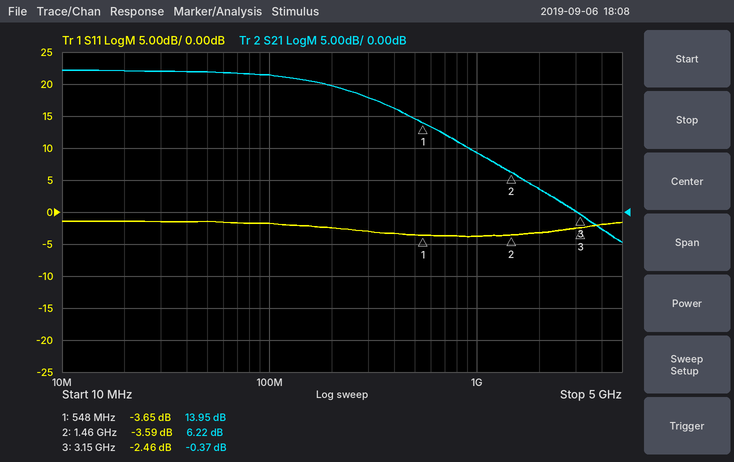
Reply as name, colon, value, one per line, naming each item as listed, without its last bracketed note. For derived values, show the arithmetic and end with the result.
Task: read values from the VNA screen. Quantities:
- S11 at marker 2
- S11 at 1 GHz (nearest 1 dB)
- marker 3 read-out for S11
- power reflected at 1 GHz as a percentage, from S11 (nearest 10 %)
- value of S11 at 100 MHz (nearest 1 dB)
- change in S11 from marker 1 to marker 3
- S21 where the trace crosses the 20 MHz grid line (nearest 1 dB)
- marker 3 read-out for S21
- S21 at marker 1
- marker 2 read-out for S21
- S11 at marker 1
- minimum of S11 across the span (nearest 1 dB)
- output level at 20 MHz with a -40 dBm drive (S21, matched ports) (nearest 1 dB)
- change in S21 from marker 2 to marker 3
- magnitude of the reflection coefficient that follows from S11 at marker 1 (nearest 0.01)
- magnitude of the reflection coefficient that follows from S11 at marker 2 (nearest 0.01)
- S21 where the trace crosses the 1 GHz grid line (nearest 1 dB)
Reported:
S11 at marker 2: -3.59 dB
S11 at 1 GHz: -4 dB
marker 3 read-out for S11: -2.46 dB
power reflected at 1 GHz as a percentage, from S11: 10^(-4/10) ≈ 40 %
value of S11 at 100 MHz: -2 dB
change in S11 from marker 1 to marker 3: -2.46 − (-3.65) = 1.19 dB
S21 where the trace crosses the 20 MHz grid line: 22 dB
marker 3 read-out for S21: -0.37 dB
S21 at marker 1: 13.95 dB
marker 2 read-out for S21: 6.22 dB
S11 at marker 1: -3.65 dB
minimum of S11 across the span: -4 dB
output level at 20 MHz with a -40 dBm drive (S21, matched ports): -40 dBm + (22 dB) = -18 dBm
change in S21 from marker 2 to marker 3: -0.37 − (6.22) = -6.59 dB
magnitude of the reflection coefficient that follows from S11 at marker 1: 10^(-3.65/20) ≈ 0.66
magnitude of the reflection coefficient that follows from S11 at marker 2: 10^(-3.59/20) ≈ 0.66
S21 where the trace crosses the 1 GHz grid line: 9 dB
